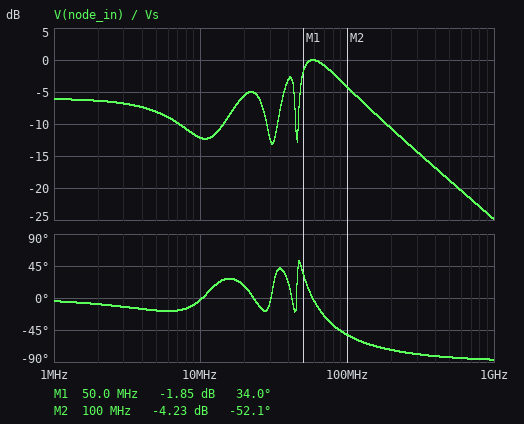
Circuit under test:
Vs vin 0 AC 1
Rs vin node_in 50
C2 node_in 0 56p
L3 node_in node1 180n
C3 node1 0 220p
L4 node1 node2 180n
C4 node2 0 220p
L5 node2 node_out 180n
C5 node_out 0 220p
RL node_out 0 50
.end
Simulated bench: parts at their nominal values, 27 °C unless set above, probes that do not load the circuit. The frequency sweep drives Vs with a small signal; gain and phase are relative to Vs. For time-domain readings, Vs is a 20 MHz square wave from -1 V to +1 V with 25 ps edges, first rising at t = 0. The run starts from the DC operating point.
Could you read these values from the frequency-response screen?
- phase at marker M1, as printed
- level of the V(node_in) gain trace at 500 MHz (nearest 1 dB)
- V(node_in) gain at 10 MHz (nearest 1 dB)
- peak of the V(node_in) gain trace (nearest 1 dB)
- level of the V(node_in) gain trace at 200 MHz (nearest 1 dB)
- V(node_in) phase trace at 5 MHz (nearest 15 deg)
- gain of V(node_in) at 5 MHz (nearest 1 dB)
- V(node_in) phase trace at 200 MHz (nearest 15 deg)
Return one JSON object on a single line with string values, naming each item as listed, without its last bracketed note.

{"phase at marker M1, as printed": "34.0 deg", "level of the V(node_in) gain trace at 500 MHz": "-19 dB", "V(node_in) gain at 10 MHz": "-12 dB", "peak of the V(node_in) gain trace": "0 dB", "level of the V(node_in) gain trace at 200 MHz": "-11 dB", "V(node_in) phase trace at 5 MHz": "-15 deg", "gain of V(node_in) at 5 MHz": "-8 dB", "V(node_in) phase trace at 200 MHz": "-75 deg"}
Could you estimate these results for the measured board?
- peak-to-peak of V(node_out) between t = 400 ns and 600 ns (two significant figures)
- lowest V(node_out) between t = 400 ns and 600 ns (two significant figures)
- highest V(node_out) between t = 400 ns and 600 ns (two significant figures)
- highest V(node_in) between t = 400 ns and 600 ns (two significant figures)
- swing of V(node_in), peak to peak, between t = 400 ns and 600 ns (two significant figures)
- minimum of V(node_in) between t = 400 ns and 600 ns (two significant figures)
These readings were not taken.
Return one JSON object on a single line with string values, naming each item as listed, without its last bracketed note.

{"peak-to-peak of V(node_out) between t = 400 ns and 600 ns": "1.2 V", "lowest V(node_out) between t = 400 ns and 600 ns": "-610 mV", "highest V(node_out) between t = 400 ns and 600 ns": "610 mV", "highest V(node_in) between t = 400 ns and 600 ns": "1.1 V", "swing of V(node_in), peak to peak, between t = 400 ns and 600 ns": "2.1 V", "minimum of V(node_in) between t = 400 ns and 600 ns": "-1.1 V"}
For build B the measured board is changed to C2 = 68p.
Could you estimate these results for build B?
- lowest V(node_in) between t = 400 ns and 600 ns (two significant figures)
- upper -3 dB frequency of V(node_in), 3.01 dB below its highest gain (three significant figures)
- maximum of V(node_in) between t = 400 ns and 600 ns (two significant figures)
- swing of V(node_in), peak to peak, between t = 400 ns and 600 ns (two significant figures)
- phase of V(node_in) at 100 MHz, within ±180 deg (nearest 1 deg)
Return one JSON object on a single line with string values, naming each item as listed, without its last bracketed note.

{"lowest V(node_in) between t = 400 ns and 600 ns": "-1.0 V", "upper -3 dB frequency of V(node_in), 3.01 dB below its highest gain": "77.4 MHz", "maximum of V(node_in) between t = 400 ns and 600 ns": "1.0 V", "swing of V(node_in), peak to peak, between t = 400 ns and 600 ns": "2.0 V", "phase of V(node_in) at 100 MHz, within ±180 deg": "-59 deg"}
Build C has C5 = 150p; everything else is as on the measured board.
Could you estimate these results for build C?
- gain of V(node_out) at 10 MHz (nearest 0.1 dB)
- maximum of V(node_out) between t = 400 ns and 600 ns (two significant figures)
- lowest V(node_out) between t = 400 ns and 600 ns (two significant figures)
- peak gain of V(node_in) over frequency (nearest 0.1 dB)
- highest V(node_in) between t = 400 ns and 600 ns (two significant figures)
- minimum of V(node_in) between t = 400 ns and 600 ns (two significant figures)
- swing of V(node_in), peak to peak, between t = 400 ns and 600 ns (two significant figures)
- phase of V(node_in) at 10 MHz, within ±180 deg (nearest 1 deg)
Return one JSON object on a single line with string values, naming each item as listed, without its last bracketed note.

{"gain of V(node_out) at 10 MHz": "-7.1 dB", "maximum of V(node_out) between t = 400 ns and 600 ns": "600 mV", "lowest V(node_out) between t = 400 ns and 600 ns": "-600 mV", "peak gain of V(node_in) over frequency": "0 dB", "highest V(node_in) between t = 400 ns and 600 ns": "1.0 V", "minimum of V(node_in) between t = 400 ns and 600 ns": "-1.0 V", "swing of V(node_in), peak to peak, between t = 400 ns and 600 ns": "2.0 V", "phase of V(node_in) at 10 MHz, within ±180 deg": "-9 deg"}
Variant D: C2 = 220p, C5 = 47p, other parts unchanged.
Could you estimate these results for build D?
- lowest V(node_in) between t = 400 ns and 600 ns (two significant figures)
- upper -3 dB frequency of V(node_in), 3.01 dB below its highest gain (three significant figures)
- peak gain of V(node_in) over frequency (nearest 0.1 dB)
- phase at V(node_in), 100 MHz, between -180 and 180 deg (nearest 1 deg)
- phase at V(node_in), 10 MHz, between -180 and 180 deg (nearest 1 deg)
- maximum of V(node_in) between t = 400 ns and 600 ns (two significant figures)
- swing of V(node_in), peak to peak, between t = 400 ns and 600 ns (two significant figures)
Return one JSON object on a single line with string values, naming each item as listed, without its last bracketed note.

{"lowest V(node_in) between t = 400 ns and 600 ns": "-490 mV", "upper -3 dB frequency of V(node_in), 3.01 dB below its highest gain": "52.1 MHz", "peak gain of V(node_in) over frequency": "-5.0 dB", "phase at V(node_in), 100 MHz, between -180 and 180 deg": "-81 deg", "phase at V(node_in), 10 MHz, between -180 and 180 deg": "-25 deg", "maximum of V(node_in) between t = 400 ns and 600 ns": "490 mV", "swing of V(node_in), peak to peak, between t = 400 ns and 600 ns": "990 mV"}
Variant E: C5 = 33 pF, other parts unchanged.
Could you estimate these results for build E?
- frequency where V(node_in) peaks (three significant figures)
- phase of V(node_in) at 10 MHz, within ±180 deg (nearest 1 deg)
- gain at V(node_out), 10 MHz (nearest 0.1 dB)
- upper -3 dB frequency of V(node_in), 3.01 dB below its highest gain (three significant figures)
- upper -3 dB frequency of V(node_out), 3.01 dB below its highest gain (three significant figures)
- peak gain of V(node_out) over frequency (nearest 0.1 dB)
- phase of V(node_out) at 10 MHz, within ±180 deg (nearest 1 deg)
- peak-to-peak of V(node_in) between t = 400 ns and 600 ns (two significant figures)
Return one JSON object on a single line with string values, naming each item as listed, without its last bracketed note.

{"frequency where V(node_in) peaks": "58.4 MHz", "phase of V(node_in) at 10 MHz, within ±180 deg": "-17 deg", "gain at V(node_out), 10 MHz": "-6.8 dB", "upper -3 dB frequency of V(node_in), 3.01 dB below its highest gain": "88.6 MHz", "upper -3 dB frequency of V(node_out), 3.01 dB below its highest gain": "44.4 MHz", "peak gain of V(node_out) over frequency": "-6.0 dB", "phase of V(node_out) at 10 MHz, within ±180 deg": "-64 deg", "peak-to-peak of V(node_in) between t = 400 ns and 600 ns": "1.8 V"}
